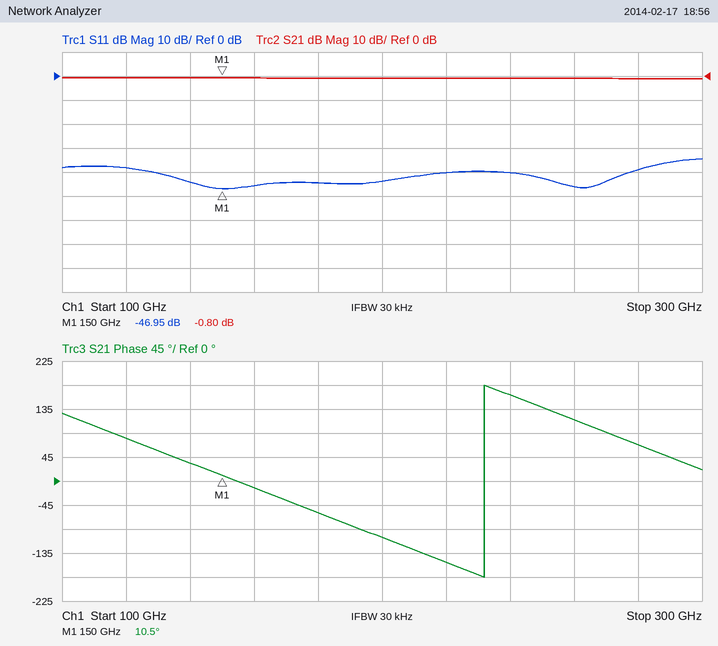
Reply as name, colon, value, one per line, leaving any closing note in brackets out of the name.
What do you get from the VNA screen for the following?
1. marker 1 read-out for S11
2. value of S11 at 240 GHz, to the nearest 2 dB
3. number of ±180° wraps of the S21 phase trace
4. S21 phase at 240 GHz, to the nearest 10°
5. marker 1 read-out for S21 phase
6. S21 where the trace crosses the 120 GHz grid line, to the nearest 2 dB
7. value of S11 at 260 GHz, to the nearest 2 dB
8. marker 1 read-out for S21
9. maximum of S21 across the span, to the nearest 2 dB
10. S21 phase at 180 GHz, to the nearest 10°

marker 1 read-out for S11: -46.95 dB
value of S11 at 240 GHz, to the nearest 2 dB: -40 dB
number of ±180° wraps of the S21 phase trace: 1
S21 phase at 240 GHz, to the nearest 10°: 160°
marker 1 read-out for S21 phase: 10.5°
S21 where the trace crosses the 120 GHz grid line, to the nearest 2 dB: 0 dB
value of S11 at 260 GHz, to the nearest 2 dB: -46 dB
marker 1 read-out for S21: -0.80 dB
maximum of S21 across the span, to the nearest 2 dB: 0 dB
S21 phase at 180 GHz, to the nearest 10°: -60°
